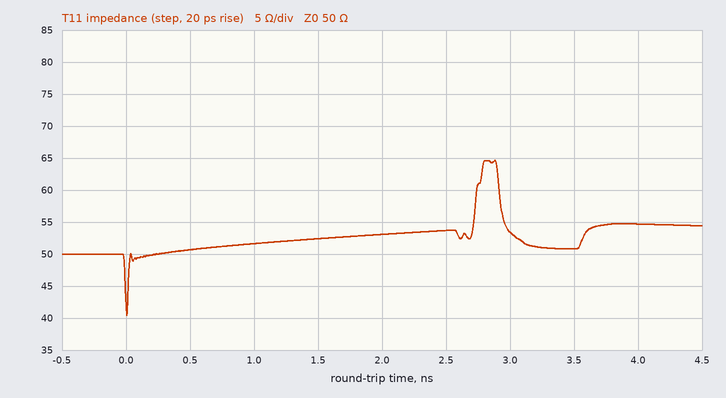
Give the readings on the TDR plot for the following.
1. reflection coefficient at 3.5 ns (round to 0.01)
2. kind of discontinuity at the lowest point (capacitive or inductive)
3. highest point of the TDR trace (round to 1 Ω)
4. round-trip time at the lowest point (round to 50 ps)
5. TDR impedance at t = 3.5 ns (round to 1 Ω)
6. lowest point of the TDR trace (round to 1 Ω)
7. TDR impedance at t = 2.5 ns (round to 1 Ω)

+0.01
capacitive
65 Ω
0 ps
51 Ω
40 Ω
54 Ω
